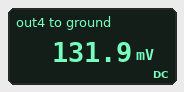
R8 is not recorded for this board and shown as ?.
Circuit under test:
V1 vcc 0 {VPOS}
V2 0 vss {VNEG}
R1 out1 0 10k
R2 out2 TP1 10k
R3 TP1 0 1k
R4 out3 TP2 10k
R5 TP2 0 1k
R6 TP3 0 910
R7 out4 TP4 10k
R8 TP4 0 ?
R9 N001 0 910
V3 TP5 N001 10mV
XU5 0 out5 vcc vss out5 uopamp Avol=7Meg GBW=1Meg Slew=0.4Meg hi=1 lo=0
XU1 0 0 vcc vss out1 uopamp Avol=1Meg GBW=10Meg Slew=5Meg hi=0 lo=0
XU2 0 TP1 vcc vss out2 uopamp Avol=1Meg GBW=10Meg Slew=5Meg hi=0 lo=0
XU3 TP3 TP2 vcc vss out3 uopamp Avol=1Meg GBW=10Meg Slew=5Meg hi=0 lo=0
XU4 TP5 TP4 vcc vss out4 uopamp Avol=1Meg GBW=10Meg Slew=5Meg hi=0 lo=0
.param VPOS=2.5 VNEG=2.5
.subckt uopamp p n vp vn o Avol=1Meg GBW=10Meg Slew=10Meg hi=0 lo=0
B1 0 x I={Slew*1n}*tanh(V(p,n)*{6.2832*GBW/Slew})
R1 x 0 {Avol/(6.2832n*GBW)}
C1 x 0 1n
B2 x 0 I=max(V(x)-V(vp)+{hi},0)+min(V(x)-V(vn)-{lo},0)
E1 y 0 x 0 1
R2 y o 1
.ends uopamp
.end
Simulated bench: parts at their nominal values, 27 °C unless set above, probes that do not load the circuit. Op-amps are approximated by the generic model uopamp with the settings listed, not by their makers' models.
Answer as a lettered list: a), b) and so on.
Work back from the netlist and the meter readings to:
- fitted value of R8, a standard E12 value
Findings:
a) 820 Ω
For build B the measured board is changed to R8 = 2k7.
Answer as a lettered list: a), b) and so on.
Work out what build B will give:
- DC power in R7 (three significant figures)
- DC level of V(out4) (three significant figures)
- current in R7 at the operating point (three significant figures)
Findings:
a) 137 nW
b) 47.0 mV
c) 3.70 µA
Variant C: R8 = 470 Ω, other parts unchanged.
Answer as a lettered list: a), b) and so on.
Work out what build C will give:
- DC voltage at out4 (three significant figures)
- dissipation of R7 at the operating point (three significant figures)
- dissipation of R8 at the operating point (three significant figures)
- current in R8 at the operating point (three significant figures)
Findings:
a) 223 mV
b) 4.53 µW
c) 213 nW
d) 21.3 µA
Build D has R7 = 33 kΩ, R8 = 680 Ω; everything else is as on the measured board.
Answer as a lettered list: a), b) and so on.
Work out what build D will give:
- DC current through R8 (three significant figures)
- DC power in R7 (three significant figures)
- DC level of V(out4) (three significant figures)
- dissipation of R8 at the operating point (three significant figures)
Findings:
a) 14.7 µA
b) 7.14 µW
c) 495 mV
d) 147 nW
